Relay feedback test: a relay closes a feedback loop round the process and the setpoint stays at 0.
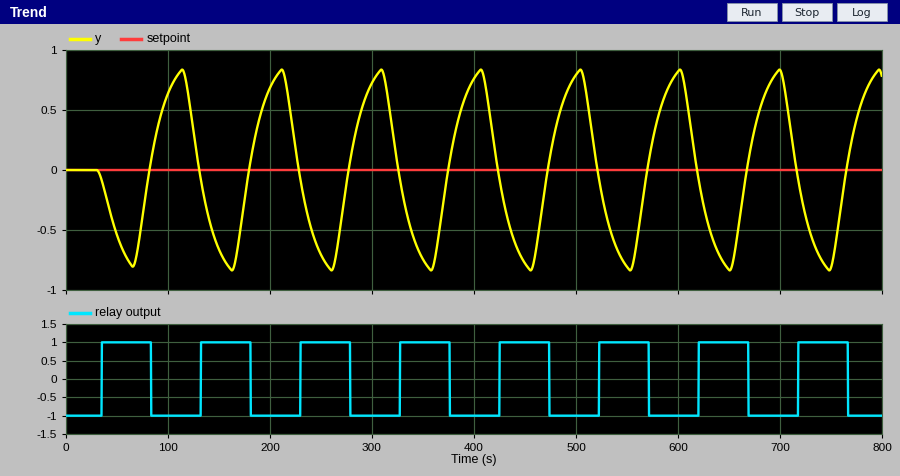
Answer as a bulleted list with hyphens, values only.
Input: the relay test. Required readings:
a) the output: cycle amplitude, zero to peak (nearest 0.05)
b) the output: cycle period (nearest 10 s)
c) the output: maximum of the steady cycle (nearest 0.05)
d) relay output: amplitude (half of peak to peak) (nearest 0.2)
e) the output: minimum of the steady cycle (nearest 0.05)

- 0.85
- 100 s
- 0.85
- 1.0
- -0.85
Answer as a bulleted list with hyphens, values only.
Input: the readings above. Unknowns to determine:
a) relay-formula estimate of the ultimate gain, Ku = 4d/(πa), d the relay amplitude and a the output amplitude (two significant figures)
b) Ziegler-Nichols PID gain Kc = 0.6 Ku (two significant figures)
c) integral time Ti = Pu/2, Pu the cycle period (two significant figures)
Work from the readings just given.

- 1.5
- 0.90
- 50 s
